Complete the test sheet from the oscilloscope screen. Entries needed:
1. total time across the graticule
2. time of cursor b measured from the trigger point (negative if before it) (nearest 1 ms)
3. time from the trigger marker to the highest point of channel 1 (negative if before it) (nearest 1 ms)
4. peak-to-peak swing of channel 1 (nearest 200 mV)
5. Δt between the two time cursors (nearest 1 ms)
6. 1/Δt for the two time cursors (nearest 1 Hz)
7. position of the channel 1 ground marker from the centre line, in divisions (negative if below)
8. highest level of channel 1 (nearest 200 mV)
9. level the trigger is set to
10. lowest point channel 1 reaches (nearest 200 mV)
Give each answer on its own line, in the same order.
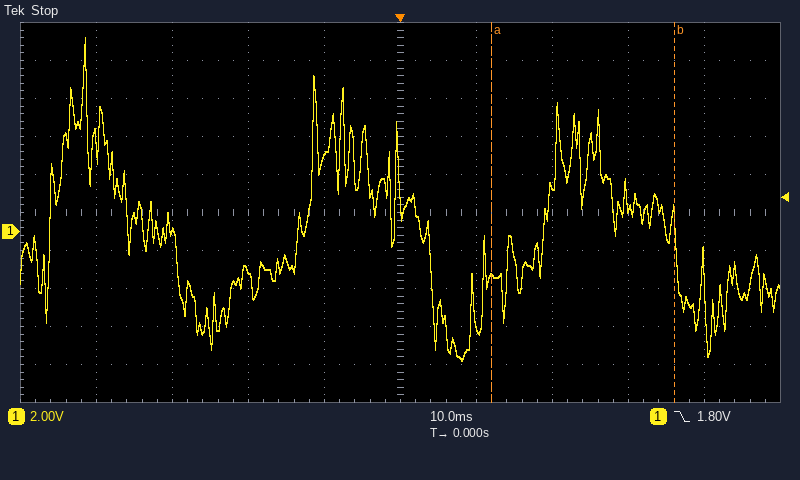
100 ms
+36 ms
-41 ms
17.0 V
24 ms
42 Hz
-0.5 div
10.2 V
1.80 V
-6.8 V
